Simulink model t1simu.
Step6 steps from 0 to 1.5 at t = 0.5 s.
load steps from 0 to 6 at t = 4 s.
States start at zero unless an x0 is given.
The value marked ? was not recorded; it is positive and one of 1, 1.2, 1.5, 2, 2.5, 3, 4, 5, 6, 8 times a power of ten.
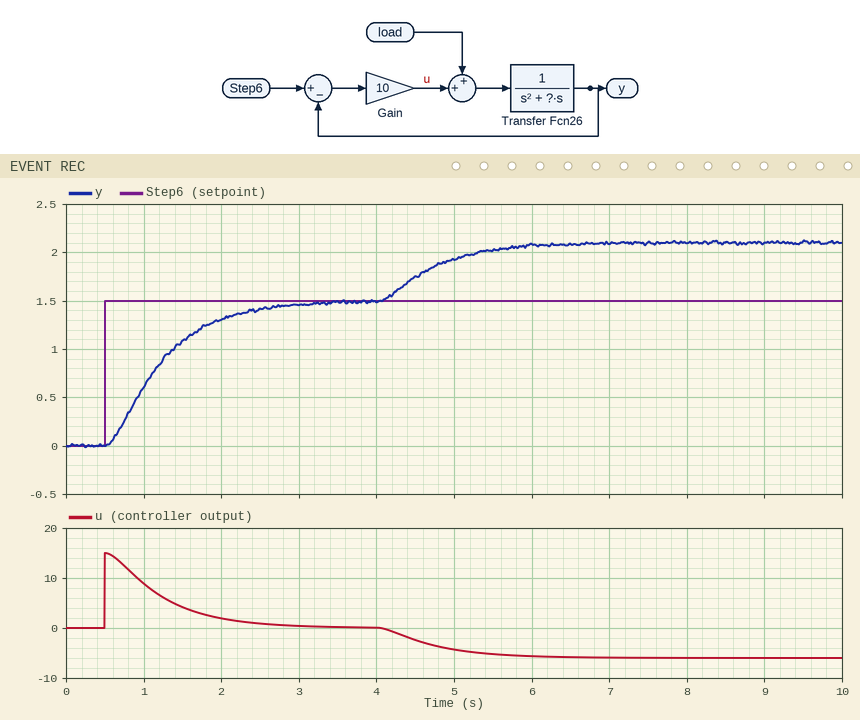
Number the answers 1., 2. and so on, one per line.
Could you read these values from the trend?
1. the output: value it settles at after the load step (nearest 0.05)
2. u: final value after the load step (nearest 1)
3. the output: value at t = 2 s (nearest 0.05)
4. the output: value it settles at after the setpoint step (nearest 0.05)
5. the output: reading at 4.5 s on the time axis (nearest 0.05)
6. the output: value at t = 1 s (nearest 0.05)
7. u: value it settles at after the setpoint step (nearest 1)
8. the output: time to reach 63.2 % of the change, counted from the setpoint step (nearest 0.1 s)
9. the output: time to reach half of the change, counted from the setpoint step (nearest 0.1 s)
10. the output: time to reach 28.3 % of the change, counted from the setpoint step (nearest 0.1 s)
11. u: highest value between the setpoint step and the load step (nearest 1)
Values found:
1. 2.10
2. -6
3. 1.30
4. 1.50
5. 1.75
6. 0.60
7. 0
8. 0.8 s
9. 0.6 s
10. 0.4 s
11. 15
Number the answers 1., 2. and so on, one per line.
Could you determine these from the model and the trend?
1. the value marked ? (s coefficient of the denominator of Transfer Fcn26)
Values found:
1. 8
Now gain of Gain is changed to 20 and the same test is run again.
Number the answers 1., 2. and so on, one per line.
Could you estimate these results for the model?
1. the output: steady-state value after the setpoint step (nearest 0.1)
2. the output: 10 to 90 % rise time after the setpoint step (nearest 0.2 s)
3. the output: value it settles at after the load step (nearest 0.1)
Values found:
1. 1.5
2. 0.6 s
3. 1.8
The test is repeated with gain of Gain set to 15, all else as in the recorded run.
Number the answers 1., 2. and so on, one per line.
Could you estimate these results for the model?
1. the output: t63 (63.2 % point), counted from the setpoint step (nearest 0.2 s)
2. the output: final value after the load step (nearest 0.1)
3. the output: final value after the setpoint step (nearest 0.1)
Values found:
1. 0.6 s
2. 1.9
3. 1.5
